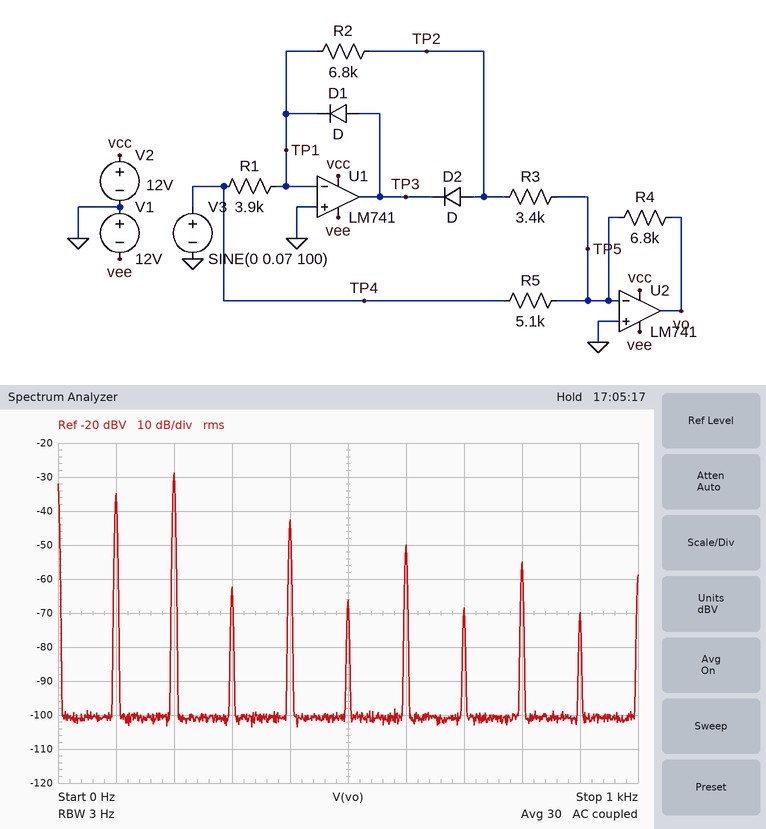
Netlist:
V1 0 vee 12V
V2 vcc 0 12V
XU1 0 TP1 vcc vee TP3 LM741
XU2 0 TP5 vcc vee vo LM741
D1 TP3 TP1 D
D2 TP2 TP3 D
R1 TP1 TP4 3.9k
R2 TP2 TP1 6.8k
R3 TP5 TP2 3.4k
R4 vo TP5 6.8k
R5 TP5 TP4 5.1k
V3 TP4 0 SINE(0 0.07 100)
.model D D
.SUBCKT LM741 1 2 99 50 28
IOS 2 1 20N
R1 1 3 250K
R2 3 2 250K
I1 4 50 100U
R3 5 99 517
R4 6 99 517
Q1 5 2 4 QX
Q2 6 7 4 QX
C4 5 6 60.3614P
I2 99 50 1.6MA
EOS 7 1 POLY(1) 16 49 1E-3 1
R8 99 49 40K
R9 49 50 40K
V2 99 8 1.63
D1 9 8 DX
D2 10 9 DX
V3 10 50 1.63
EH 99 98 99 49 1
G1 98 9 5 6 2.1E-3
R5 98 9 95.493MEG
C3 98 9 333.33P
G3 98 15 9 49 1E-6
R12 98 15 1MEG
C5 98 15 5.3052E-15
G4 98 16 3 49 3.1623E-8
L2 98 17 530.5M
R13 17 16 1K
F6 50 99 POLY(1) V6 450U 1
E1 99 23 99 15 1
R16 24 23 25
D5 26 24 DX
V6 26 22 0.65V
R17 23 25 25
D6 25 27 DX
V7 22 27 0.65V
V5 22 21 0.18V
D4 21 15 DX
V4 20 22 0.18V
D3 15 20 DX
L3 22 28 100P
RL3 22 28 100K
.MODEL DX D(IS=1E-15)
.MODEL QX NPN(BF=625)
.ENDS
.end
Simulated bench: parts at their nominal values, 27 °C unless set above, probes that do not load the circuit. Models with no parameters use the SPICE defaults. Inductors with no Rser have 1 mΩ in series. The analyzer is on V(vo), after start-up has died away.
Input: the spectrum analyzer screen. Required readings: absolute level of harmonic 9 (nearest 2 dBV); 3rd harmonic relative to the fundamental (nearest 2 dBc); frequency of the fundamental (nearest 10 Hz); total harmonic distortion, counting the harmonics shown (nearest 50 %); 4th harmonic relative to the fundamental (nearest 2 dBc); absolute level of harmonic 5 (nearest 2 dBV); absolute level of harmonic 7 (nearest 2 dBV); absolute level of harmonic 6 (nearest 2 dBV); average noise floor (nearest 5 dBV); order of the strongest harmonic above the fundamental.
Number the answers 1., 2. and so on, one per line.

1. -70 dBV
2. -28 dBc
3. 100 Hz
4. 200 %
5. -8 dBc
6. -66 dBV
7. -68 dBV
8. -50 dBV
9. -100 dBV
10. 2
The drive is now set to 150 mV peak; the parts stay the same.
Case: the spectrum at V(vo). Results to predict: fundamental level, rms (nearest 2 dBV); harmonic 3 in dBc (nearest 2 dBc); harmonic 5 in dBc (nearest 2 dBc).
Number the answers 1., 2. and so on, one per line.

1. -28 dBV
2. -34 dBc
3. -38 dBc
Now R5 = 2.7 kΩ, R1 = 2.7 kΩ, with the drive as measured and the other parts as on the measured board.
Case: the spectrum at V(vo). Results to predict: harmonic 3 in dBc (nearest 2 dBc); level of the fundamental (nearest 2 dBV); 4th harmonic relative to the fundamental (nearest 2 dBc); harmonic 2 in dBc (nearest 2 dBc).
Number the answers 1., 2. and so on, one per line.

1. -10 dBc
2. -50 dBV
3. 12 dBc
4. 26 dBc
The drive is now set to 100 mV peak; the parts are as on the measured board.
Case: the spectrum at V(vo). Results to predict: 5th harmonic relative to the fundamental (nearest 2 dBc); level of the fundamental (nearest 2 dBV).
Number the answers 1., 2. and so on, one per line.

1. -34 dBc
2. -32 dBV
